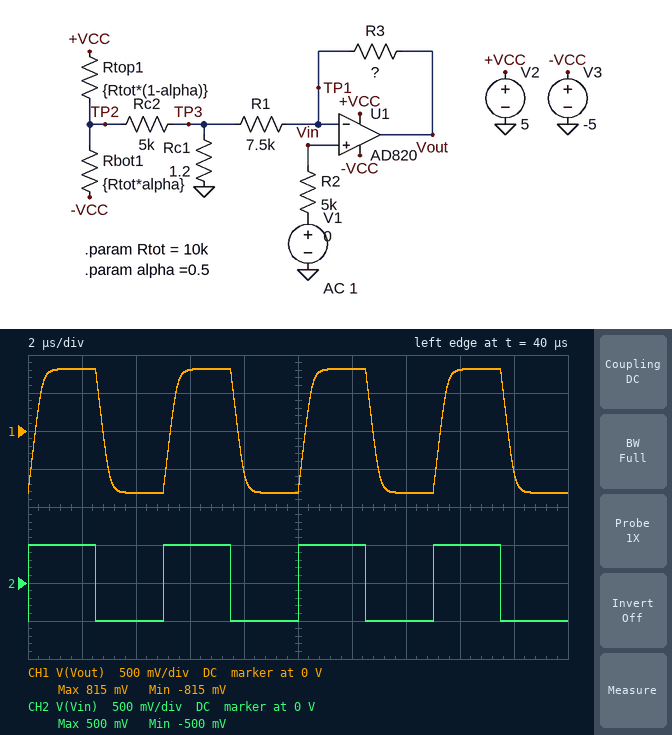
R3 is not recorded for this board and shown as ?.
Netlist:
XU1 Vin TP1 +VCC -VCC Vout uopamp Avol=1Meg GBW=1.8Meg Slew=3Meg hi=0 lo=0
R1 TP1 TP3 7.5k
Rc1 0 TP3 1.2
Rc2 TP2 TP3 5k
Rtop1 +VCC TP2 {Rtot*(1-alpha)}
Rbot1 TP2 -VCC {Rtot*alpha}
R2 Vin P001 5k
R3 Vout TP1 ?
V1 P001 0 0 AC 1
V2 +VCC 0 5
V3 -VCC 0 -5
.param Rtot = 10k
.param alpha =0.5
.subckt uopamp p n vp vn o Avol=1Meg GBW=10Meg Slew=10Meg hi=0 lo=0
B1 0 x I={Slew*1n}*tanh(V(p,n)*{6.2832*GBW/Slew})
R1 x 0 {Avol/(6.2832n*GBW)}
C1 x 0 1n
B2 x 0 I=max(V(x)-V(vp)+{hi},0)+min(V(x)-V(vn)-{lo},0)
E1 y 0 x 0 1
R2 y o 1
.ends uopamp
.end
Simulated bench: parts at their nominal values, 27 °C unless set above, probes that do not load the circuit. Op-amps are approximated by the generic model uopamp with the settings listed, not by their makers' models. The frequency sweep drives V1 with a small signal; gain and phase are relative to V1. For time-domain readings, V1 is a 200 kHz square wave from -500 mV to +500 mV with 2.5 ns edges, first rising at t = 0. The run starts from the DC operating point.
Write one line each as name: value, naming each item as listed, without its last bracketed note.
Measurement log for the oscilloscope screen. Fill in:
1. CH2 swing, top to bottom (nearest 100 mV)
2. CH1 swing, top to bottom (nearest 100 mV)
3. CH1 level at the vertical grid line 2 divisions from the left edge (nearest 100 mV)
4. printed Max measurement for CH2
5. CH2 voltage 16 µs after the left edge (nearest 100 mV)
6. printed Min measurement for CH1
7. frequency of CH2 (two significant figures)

CH2 swing, top to bottom: 1.0 V
CH1 swing, top to bottom: 1.6 V
CH1 level at the vertical grid line 2 divisions from the left edge: -800 mV
printed Max measurement for CH2: 500 mV
CH2 voltage 16 µs after the left edge: 500 mV
printed Min measurement for CH1: -815 mV
frequency of CH2: 200 kHz
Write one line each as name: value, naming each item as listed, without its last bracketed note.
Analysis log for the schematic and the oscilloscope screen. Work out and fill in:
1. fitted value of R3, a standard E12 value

fitted value of R3, a standard E12 value: 4.7 kΩ
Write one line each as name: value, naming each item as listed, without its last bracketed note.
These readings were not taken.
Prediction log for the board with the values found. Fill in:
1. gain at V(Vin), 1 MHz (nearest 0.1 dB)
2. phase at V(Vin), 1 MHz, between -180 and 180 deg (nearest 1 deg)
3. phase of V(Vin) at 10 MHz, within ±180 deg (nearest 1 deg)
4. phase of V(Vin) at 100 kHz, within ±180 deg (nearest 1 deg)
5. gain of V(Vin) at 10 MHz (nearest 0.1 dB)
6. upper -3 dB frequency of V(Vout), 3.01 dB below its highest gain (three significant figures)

gain at V(Vin), 1 MHz: 0 dB
phase at V(Vin), 1 MHz, between -180 and 180 deg: 0 deg
phase of V(Vin) at 10 MHz, within ±180 deg: 0 deg
phase of V(Vin) at 100 kHz, within ±180 deg: 0 deg
gain of V(Vin) at 10 MHz: 0 dB
upper -3 dB frequency of V(Vout), 3.01 dB below its highest gain: 1.11 MHz
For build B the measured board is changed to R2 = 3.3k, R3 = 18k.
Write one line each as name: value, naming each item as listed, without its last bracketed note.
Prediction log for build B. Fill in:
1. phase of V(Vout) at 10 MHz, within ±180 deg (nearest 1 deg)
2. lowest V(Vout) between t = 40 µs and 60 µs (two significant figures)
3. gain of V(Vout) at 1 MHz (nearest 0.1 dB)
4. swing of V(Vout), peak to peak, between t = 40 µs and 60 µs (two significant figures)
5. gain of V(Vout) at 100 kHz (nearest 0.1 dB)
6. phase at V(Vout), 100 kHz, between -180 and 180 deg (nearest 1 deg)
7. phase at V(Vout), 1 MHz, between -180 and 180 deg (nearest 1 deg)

phase of V(Vout) at 10 MHz, within ±180 deg: -87 deg
lowest V(Vout) between t = 40 µs and 60 µs: -1.7 V
gain of V(Vout) at 1 MHz: 4.0 dB
swing of V(Vout), peak to peak, between t = 40 µs and 60 µs: 3.4 V
gain of V(Vout) at 100 kHz: 10.5 dB
phase at V(Vout), 100 kHz, between -180 and 180 deg: -11 deg
phase at V(Vout), 1 MHz, between -180 and 180 deg: -62 deg
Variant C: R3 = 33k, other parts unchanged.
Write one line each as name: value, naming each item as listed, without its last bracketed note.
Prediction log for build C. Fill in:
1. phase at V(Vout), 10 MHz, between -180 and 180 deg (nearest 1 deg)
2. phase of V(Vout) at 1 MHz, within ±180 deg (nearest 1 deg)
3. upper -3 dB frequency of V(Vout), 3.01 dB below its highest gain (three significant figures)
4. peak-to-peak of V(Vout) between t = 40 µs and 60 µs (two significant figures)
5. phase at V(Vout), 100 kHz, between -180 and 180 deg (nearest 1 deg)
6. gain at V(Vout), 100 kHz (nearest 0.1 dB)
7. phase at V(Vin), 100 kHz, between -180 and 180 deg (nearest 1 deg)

phase at V(Vout), 10 MHz, between -180 and 180 deg: -88 deg
phase of V(Vout) at 1 MHz, within ±180 deg: -72 deg
upper -3 dB frequency of V(Vout), 3.01 dB below its highest gain: 333 kHz
peak-to-peak of V(Vout) between t = 40 µs and 60 µs: 5.1 V
phase at V(Vout), 100 kHz, between -180 and 180 deg: -17 deg
gain at V(Vout), 100 kHz: 14.3 dB
phase at V(Vin), 100 kHz, between -180 and 180 deg: 0 deg
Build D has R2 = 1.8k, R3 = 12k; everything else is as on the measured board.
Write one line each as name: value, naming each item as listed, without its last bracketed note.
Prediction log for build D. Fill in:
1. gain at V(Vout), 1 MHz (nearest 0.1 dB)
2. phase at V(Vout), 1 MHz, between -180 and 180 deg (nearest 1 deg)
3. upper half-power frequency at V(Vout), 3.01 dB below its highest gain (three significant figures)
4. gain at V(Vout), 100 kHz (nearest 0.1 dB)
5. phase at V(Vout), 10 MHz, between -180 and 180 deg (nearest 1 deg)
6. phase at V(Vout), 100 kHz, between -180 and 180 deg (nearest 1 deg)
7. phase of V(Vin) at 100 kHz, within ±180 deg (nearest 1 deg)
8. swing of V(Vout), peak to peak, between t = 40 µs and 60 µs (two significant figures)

gain at V(Vout), 1 MHz: 3.4 dB
phase at V(Vout), 1 MHz, between -180 and 180 deg: -55 deg
upper half-power frequency at V(Vout), 3.01 dB below its highest gain: 692 kHz
gain at V(Vout), 100 kHz: 8.2 dB
phase at V(Vout), 10 MHz, between -180 and 180 deg: -86 deg
phase at V(Vout), 100 kHz, between -180 and 180 deg: -8 deg
phase of V(Vin) at 100 kHz, within ±180 deg: 0 deg
swing of V(Vout), peak to peak, between t = 40 µs and 60 µs: 2.6 V
